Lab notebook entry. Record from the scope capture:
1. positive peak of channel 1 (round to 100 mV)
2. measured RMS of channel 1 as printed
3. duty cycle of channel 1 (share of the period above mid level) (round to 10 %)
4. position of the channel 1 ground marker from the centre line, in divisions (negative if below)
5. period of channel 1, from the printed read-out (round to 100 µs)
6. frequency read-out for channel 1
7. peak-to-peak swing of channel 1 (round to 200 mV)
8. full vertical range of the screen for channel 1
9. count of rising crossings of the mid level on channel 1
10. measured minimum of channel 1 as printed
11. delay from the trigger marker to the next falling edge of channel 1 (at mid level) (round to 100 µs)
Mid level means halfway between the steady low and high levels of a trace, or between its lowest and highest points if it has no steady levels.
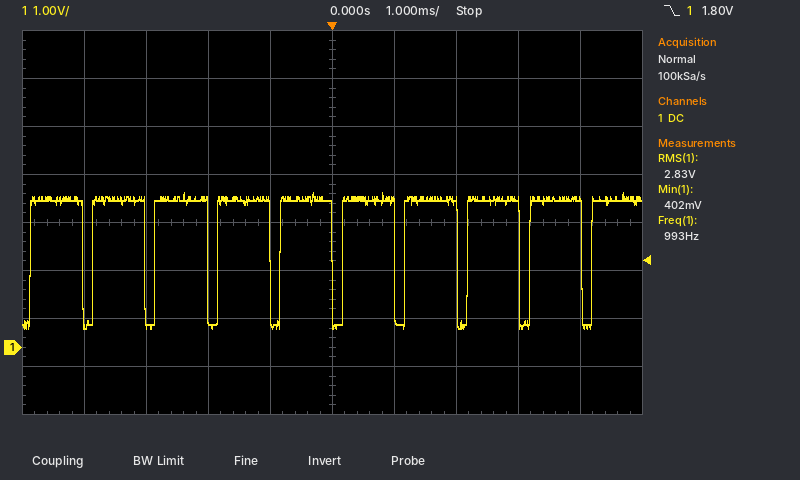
3.2 V
2.83 V
80 %
-2.6 div
1.0 ms
993 Hz
2.8 V
8 V
10
402 mV
1.0 ms
